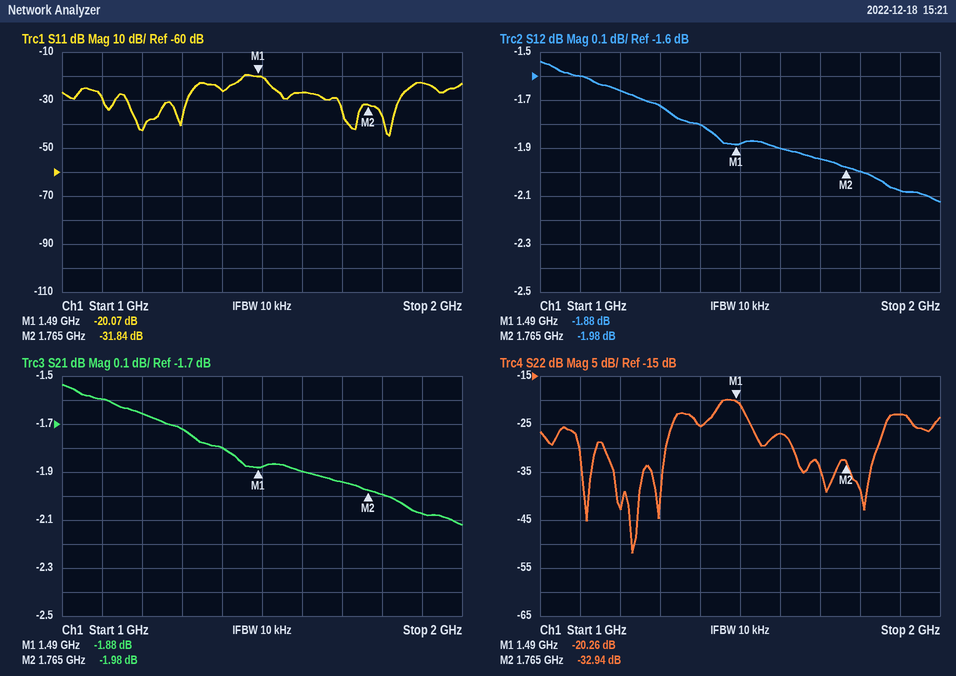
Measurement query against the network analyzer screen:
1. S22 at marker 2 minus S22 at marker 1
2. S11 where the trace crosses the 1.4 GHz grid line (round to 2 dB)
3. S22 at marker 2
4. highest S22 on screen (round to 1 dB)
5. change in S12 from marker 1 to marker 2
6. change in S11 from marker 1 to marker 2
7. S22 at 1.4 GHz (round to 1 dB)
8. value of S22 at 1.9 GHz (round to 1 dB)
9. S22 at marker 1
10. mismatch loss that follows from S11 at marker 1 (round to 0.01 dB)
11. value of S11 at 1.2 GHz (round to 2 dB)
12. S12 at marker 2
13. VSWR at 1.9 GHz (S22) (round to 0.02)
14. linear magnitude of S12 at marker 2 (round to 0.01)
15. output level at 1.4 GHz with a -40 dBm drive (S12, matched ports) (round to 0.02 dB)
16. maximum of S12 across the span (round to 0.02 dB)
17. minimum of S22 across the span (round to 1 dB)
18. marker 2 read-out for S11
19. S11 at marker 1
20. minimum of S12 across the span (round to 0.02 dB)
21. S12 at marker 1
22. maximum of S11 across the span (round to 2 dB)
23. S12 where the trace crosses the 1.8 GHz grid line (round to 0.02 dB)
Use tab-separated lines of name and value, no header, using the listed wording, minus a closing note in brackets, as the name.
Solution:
S22 at marker 2 minus S22 at marker 1	-12.68 dB
S11 where the trace crosses the 1.4 GHz grid line	-26 dB
S22 at marker 2	-32.94 dB
highest S22 on screen	-20 dB
change in S12 from marker 1 to marker 2	-0.10 dB
change in S11 from marker 1 to marker 2	-11.77 dB
S22 at 1.4 GHz	-25 dB
value of S22 at 1.9 GHz	-23 dB
S22 at marker 1	-20.26 dB
mismatch loss that follows from S11 at marker 1	0.04 dB
value of S11 at 1.2 GHz	-42 dB
S12 at marker 2	-1.98 dB
VSWR at 1.9 GHz (S22)	1.16
linear magnitude of S12 at marker 2	0.80
output level at 1.4 GHz with a -40 dBm drive (S12, matched ports)	-41.80 dBm
maximum of S12 across the span	-1.54 dB
minimum of S22 across the span	-52 dB
marker 2 read-out for S11	-31.84 dB
S11 at marker 1	-20.07 dB
minimum of S12 across the span	-2.12 dB
S12 at marker 1	-1.88 dB
maximum of S11 across the span	-20 dB
S12 where the trace crosses the 1.8 GHz grid line	-2.00 dB
